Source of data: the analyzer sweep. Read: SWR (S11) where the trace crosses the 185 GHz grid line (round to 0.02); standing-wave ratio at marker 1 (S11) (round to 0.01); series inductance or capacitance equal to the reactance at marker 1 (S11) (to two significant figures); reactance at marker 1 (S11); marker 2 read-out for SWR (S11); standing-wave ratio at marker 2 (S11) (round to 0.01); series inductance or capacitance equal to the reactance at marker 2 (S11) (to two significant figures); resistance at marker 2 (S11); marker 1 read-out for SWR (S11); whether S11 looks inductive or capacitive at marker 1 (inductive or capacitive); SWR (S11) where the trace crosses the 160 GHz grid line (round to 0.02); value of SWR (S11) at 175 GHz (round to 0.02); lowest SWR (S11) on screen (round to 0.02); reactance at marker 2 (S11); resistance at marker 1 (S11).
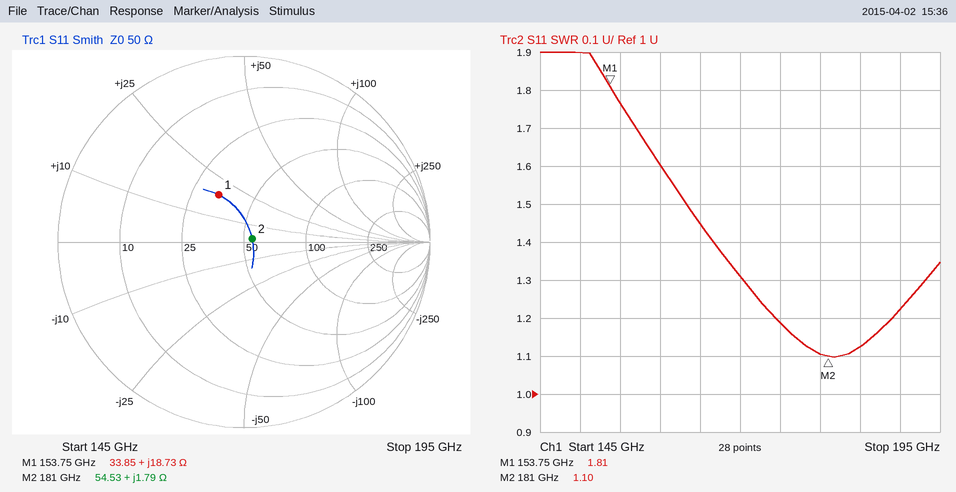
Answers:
1.12
1.81
19 pH
+18.73 Ω
1.10
1.10
1.6 pH
54.53 Ω
1.81
inductive
1.60
1.18
1.10
+1.79 Ω
33.85 Ω
